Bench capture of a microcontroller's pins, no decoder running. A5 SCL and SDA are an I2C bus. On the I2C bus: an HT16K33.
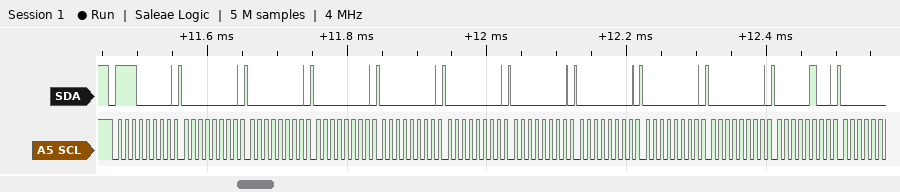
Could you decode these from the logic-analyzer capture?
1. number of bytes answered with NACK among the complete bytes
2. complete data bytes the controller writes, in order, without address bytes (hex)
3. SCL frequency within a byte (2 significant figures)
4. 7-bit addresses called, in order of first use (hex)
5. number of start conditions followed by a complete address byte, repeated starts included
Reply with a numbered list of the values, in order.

1. 0
2. 00 00 00 00 00 00 00 00 00 04
3. 100 kHz
4. 0x70
5. 1
